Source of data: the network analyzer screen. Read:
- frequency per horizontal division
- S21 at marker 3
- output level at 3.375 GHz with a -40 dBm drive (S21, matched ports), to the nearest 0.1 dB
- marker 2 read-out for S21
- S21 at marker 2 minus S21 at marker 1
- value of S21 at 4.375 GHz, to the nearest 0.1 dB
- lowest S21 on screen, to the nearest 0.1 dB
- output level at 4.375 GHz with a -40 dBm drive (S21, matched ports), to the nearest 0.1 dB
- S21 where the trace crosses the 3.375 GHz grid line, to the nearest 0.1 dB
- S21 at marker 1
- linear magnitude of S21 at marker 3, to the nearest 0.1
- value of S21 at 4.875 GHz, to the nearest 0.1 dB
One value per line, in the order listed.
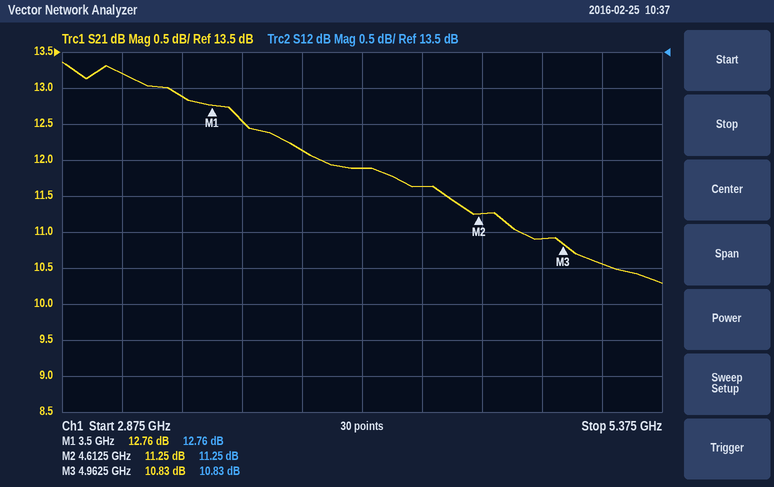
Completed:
250 MHz
10.83 dB
-27.1 dBm
11.25 dB
-1.51 dB
11.6 dB
10.3 dB
-28.4 dBm
12.9 dB
12.76 dB
3.5
10.9 dB
